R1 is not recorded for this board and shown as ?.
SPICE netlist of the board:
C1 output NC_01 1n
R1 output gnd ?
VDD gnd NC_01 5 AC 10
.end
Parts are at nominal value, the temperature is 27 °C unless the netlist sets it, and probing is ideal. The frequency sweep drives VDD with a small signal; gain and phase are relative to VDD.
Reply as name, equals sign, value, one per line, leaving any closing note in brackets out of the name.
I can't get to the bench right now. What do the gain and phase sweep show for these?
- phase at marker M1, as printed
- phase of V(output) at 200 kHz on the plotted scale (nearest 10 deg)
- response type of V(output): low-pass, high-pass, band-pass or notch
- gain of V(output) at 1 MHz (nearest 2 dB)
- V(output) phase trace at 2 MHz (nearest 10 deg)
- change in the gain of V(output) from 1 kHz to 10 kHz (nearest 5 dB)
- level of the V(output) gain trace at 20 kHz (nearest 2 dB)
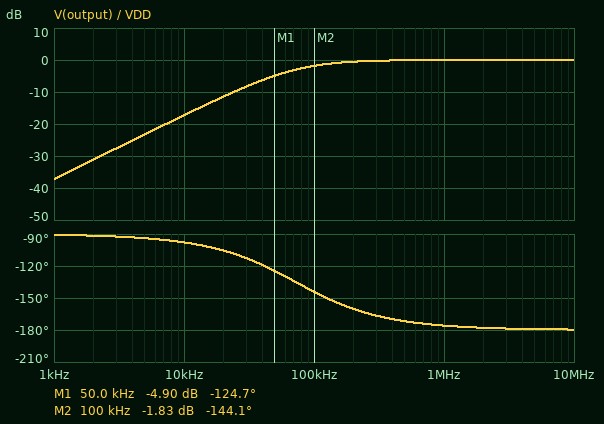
phase at marker M1, as printed = -124.7 deg
phase of V(output) at 200 kHz on the plotted scale = -160 deg
response type of V(output): low-pass, high-pass, band-pass or notch = high-pass
gain of V(output) at 1 MHz = 0 dB
V(output) phase trace at 2 MHz = -180 deg
change in the gain of V(output) from 1 kHz to 10 kHz = 20 dB
level of the V(output) gain trace at 20 kHz = -12 dB
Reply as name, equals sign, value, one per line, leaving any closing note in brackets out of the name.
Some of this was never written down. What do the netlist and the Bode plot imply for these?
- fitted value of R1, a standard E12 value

fitted value of R1, a standard E12 value = 2.2 kΩ
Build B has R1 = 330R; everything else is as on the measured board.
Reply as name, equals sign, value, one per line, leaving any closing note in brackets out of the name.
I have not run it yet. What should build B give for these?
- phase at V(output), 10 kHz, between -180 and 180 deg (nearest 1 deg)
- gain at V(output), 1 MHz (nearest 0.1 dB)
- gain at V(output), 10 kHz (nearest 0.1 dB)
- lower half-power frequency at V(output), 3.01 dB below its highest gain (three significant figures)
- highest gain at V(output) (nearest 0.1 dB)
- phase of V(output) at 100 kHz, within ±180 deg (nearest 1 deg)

phase at V(output), 10 kHz, between -180 and 180 deg = -91 deg
gain at V(output), 1 MHz = -0.9 dB
gain at V(output), 10 kHz = -33.7 dB
lower half-power frequency at V(output), 3.01 dB below its highest gain = 482 kHz
highest gain at V(output) = 0 dB
phase of V(output) at 100 kHz, within ±180 deg = -102 deg
